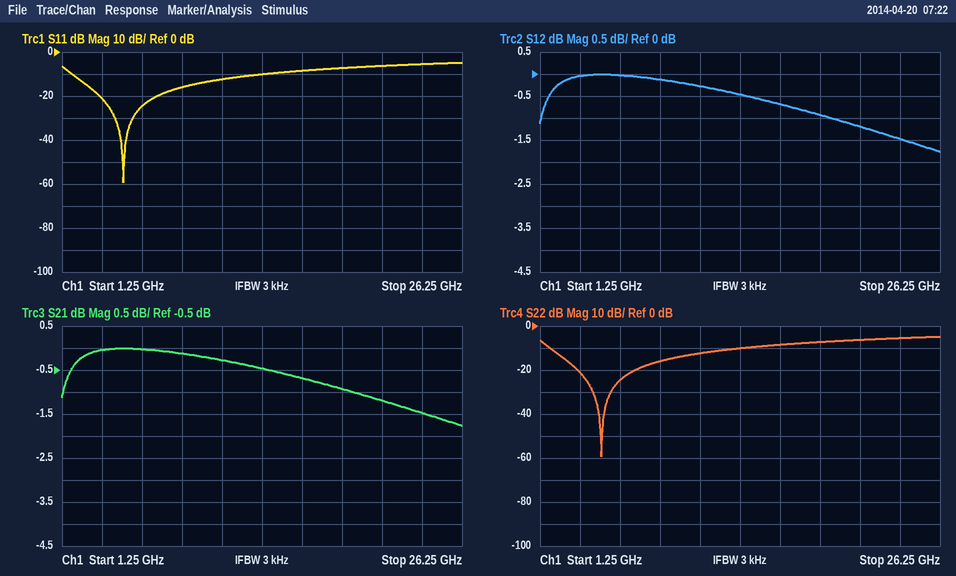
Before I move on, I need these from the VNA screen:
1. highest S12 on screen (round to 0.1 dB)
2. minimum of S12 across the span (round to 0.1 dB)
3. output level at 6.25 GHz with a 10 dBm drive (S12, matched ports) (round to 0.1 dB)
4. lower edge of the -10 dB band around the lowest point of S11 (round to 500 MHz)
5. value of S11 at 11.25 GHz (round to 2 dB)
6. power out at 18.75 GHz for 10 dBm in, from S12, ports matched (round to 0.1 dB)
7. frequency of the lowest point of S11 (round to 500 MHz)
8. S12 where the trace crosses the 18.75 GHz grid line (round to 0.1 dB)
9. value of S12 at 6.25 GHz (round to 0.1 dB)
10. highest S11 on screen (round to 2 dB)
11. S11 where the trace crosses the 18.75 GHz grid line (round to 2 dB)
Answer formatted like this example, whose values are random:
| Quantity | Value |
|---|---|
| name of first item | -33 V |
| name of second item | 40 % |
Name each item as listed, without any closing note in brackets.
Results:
| Quantity | Value |
|---|---|
| highest S12 on screen | 0.0 dB |
| minimum of S12 across the span | -1.8 dB |
| output level at 6.25 GHz with a 10 dBm drive (S12, matched ports) | 10.0 dBm |
| lower edge of the -10 dB band around the lowest point of S11 | 2.0 GHz |
| value of S11 at 11.25 GHz | -12 dB |
| power out at 18.75 GHz for 10 dBm in, from S12, ports matched | 9.1 dBm |
| frequency of the lowest point of S11 | 5.0 GHz |
| S12 where the trace crosses the 18.75 GHz grid line | -0.9 dB |
| value of S12 at 6.25 GHz | 0.0 dB |
| highest S11 on screen | -4 dB |
| S11 where the trace crosses the 18.75 GHz grid line | -8 dB |
